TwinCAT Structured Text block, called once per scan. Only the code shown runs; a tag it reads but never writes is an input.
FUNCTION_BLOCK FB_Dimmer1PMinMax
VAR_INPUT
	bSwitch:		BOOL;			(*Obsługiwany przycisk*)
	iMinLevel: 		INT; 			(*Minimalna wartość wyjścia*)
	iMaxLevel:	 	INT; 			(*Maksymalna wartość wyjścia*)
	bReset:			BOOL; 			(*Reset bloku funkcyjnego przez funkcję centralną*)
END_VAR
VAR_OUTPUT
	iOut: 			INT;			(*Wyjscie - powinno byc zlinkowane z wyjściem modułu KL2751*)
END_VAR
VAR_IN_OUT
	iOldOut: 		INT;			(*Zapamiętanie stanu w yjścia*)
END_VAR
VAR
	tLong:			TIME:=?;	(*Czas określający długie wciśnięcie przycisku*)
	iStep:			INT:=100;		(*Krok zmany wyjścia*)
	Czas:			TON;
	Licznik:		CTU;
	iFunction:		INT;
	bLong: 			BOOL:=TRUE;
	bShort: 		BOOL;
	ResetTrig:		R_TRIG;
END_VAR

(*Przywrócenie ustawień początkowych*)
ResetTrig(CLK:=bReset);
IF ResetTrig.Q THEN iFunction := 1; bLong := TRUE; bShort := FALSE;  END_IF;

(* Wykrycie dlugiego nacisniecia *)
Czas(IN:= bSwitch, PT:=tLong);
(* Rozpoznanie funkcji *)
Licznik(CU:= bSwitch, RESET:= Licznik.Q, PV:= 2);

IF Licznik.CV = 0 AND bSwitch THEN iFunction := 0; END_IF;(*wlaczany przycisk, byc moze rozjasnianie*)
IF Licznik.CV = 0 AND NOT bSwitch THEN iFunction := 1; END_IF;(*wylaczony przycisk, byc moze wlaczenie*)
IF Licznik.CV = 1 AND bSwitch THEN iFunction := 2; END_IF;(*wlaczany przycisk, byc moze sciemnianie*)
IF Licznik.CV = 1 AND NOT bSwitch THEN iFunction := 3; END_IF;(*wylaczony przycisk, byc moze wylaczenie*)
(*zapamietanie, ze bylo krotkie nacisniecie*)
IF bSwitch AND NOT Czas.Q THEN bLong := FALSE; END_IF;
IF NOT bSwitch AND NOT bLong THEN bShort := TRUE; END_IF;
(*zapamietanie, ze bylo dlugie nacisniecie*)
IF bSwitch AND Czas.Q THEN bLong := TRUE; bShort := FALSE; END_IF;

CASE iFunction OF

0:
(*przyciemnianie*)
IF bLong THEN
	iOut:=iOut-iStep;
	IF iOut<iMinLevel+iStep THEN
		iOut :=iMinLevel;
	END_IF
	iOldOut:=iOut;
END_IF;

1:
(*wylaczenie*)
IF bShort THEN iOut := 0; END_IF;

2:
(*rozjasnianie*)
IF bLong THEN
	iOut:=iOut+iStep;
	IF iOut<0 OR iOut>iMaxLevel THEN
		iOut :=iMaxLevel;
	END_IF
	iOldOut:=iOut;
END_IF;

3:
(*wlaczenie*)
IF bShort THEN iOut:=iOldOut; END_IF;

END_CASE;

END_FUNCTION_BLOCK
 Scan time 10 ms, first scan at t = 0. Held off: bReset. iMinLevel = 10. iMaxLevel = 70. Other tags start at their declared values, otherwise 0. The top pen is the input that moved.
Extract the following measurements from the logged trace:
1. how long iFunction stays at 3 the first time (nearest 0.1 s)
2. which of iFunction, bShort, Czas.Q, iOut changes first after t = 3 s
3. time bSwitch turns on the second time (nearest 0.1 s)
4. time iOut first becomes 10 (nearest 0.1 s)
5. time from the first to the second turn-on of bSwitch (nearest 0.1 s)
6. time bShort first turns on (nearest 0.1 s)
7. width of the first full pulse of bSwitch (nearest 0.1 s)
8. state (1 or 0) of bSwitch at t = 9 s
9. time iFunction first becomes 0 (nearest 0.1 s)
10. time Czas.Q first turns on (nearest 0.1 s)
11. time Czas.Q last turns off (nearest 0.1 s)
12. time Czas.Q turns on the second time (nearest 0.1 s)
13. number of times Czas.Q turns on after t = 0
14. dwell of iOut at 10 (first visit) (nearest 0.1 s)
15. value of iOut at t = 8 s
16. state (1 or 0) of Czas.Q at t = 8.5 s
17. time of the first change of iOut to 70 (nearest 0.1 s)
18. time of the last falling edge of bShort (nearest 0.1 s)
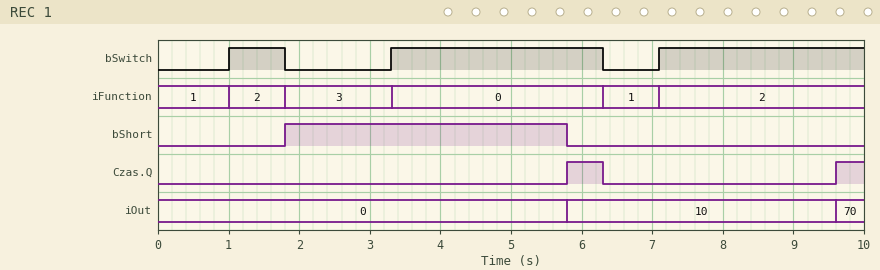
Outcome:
1.5 s
iFunction
3.3 s
5.8 s
2.3 s
1.8 s
0.8 s
1
3.3 s
5.8 s
6.3 s
9.6 s
2
3.8 s
10
0
9.6 s
5.8 s
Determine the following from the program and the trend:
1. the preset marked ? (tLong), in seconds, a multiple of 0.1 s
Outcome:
2.5 s
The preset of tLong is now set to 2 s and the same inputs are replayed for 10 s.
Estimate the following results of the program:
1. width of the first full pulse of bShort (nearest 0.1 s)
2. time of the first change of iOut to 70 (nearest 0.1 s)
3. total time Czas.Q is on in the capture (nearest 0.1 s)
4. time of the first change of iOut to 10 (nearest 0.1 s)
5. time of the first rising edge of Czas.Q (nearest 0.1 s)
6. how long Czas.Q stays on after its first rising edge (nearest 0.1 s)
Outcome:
3.5 s
9.1 s
1.9 s
5.3 s
5.3 s
1.0 s
